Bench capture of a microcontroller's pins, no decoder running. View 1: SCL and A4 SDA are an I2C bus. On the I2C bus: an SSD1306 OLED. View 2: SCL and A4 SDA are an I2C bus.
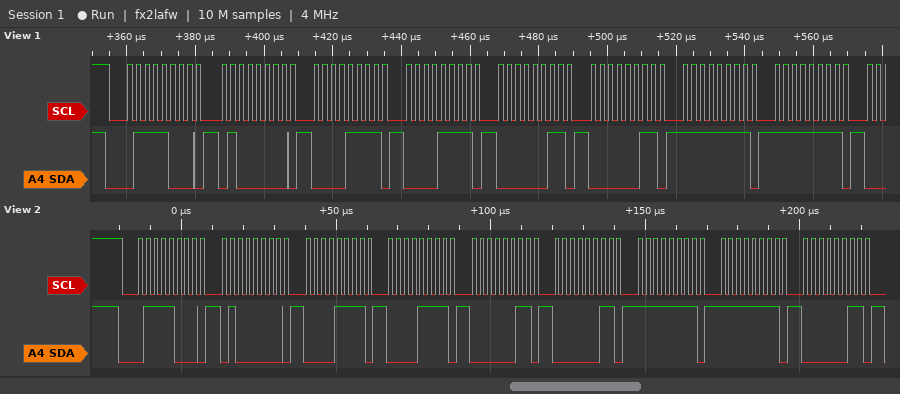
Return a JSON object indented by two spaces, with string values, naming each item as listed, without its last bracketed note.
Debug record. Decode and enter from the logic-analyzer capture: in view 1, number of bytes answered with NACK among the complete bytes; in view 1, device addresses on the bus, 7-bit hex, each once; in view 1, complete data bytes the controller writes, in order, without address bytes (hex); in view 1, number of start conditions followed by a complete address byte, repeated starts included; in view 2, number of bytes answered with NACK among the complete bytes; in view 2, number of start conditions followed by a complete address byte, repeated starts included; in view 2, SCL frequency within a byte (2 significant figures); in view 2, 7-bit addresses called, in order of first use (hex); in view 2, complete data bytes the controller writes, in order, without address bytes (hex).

{
  "in view 1, number of bytes answered with NACK among the complete bytes": "0",
  "in view 1, device addresses on the bus, 7-bit hex, each once": "0x3C",
  "in view 1, complete data bytes the controller writes, in order, without address bytes": "40 0F 0F 03 03 FF FF",
  "in view 1, number of start conditions followed by a complete address byte, repeated starts included": "1",
  "in view 2, number of bytes answered with NACK among the complete bytes": "0",
  "in view 2, number of start conditions followed by a complete address byte, repeated starts included": "1",
  "in view 2, SCL frequency within a byte": "400 kHz",
  "in view 2, 7-bit addresses called, in order of first use": "0x3C",
  "in view 2, complete data bytes the controller writes, in order, without address bytes": "40 0F 0F 03 03 FF FF 03"
}
